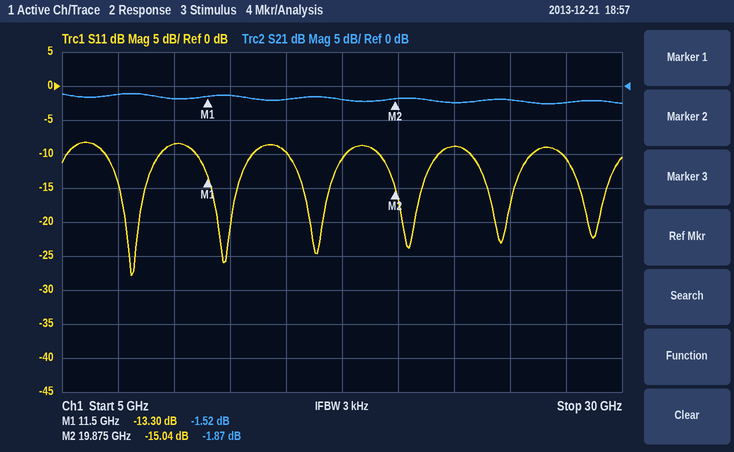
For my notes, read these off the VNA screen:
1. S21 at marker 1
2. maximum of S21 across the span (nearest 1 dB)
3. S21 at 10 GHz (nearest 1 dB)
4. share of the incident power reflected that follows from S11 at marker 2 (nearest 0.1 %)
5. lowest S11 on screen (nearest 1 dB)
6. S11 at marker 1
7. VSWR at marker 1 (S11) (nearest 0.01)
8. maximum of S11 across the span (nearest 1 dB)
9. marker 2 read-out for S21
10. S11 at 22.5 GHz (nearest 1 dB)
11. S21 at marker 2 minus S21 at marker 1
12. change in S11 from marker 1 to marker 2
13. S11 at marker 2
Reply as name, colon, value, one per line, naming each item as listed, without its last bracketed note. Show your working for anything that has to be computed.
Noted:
S21 at marker 1: -1.52 dB
maximum of S21 across the span: -1 dB
S21 at 10 GHz: -2 dB
share of the incident power reflected that follows from S11 at marker 2: 10^(-15.04/10) ≈ 3.1 %
lowest S11 on screen: -28 dB
S11 at marker 1: -13.30 dB
VSWR at marker 1 (S11): (1 + 0.2163)/(1 − 0.2163) ≈ 1.55
maximum of S11 across the span: -8 dB
marker 2 read-out for S21: -1.87 dB
S11 at 22.5 GHz: -9 dB
S21 at marker 2 minus S21 at marker 1: -1.87 − (-1.52) = -0.35 dB
change in S11 from marker 1 to marker 2: -15.04 − (-13.3) = -1.74 dB
S11 at marker 2: -15.04 dB
